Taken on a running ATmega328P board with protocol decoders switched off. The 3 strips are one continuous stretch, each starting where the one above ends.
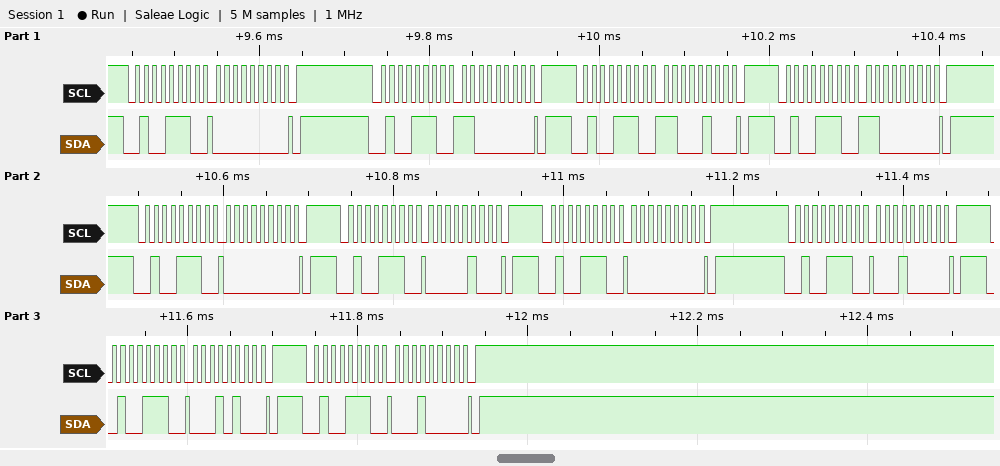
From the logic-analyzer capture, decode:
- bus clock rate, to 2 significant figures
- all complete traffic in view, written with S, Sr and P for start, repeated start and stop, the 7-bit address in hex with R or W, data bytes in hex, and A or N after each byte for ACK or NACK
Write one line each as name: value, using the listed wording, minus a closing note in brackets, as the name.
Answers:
bus clock rate, to 2 significant figures: 100 kHz
all complete traffic in view, written with S, Sr and P for start, repeated start and stop, the 7-bit address in hex with R or W, data bytes in hex, and A or N after each byte for ACK or NACK: S 27W A 00 A P S 27W A C0 A P S 27W A C4 A P S 27W A C0 A P S 27W A 00 A P S 27W A 04 A P S 27W A 00 A P S 27W A 10 A P S 27W A 14 A P S 27W A 10 A P
